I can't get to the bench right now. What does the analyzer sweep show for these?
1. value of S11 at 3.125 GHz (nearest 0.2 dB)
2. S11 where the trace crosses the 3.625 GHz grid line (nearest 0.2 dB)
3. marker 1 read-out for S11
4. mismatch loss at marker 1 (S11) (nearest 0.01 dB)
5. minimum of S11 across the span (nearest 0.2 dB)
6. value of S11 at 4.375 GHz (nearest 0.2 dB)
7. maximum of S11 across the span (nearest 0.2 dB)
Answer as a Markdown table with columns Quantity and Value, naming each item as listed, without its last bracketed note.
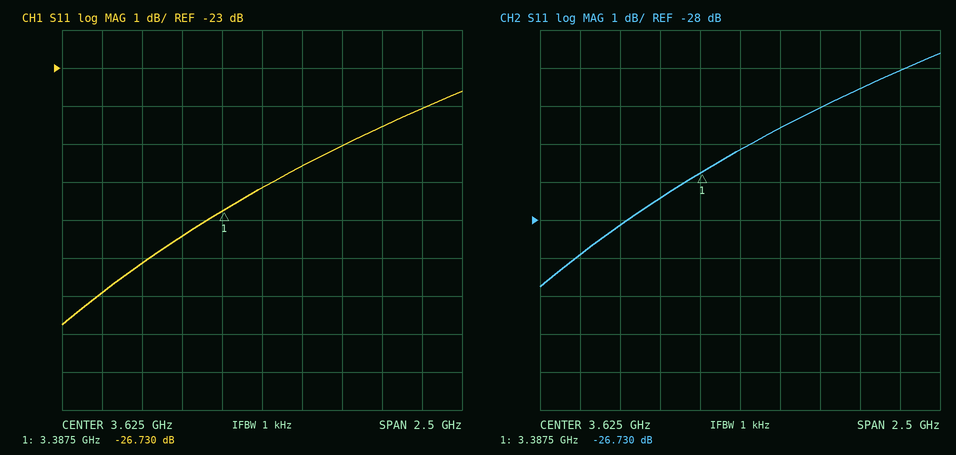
| Quantity | Value |
|---|---|
| value of S11 at 3.125 GHz | -27.4 dB |
| S11 where the trace crosses the 3.625 GHz grid line | -26.2 dB |
| marker 1 read-out for S11 | -26.730 dB |
| mismatch loss at marker 1 (S11) | 0.01 dB |
| minimum of S11 across the span | -29.8 dB |
| value of S11 at 4.375 GHz | -24.6 dB |
| maximum of S11 across the span | -23.6 dB |
